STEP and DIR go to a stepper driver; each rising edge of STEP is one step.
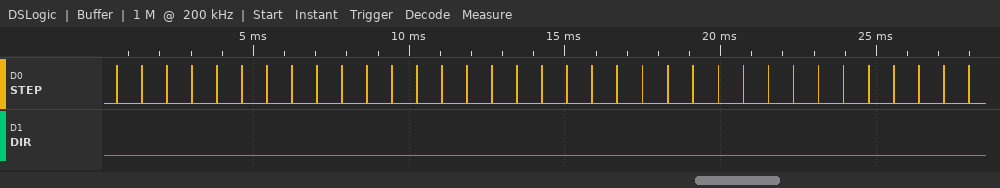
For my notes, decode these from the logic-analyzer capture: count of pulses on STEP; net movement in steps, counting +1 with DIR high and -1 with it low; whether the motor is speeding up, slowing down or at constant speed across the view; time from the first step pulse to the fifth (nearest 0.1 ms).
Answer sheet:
35
-35
constant speed
3.2 ms
